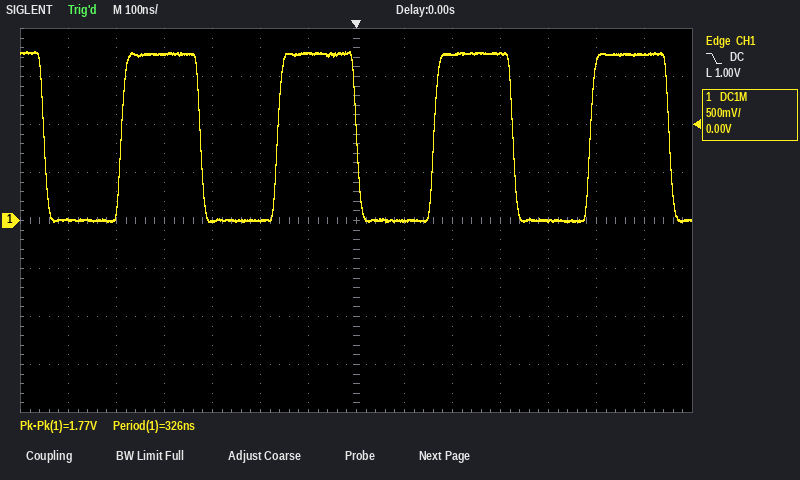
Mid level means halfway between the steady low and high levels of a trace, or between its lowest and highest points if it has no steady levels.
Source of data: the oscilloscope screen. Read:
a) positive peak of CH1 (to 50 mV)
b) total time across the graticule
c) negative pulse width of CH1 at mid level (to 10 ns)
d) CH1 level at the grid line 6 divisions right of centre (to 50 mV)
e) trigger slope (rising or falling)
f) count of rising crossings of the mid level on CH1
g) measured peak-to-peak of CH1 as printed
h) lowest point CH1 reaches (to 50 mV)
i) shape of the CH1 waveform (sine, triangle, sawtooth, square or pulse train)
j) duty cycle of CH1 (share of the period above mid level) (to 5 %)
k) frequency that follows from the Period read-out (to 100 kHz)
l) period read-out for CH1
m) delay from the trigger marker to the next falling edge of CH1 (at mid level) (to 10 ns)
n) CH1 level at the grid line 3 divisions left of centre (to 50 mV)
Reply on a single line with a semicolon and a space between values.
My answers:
1.75 V; 1.4 µs; 160 ns; 1.75 V; falling; 4; 1.77 V; 0 mV; square; 50 %; 3.1 MHz; 326 ns; 330 ns; 0 mV
